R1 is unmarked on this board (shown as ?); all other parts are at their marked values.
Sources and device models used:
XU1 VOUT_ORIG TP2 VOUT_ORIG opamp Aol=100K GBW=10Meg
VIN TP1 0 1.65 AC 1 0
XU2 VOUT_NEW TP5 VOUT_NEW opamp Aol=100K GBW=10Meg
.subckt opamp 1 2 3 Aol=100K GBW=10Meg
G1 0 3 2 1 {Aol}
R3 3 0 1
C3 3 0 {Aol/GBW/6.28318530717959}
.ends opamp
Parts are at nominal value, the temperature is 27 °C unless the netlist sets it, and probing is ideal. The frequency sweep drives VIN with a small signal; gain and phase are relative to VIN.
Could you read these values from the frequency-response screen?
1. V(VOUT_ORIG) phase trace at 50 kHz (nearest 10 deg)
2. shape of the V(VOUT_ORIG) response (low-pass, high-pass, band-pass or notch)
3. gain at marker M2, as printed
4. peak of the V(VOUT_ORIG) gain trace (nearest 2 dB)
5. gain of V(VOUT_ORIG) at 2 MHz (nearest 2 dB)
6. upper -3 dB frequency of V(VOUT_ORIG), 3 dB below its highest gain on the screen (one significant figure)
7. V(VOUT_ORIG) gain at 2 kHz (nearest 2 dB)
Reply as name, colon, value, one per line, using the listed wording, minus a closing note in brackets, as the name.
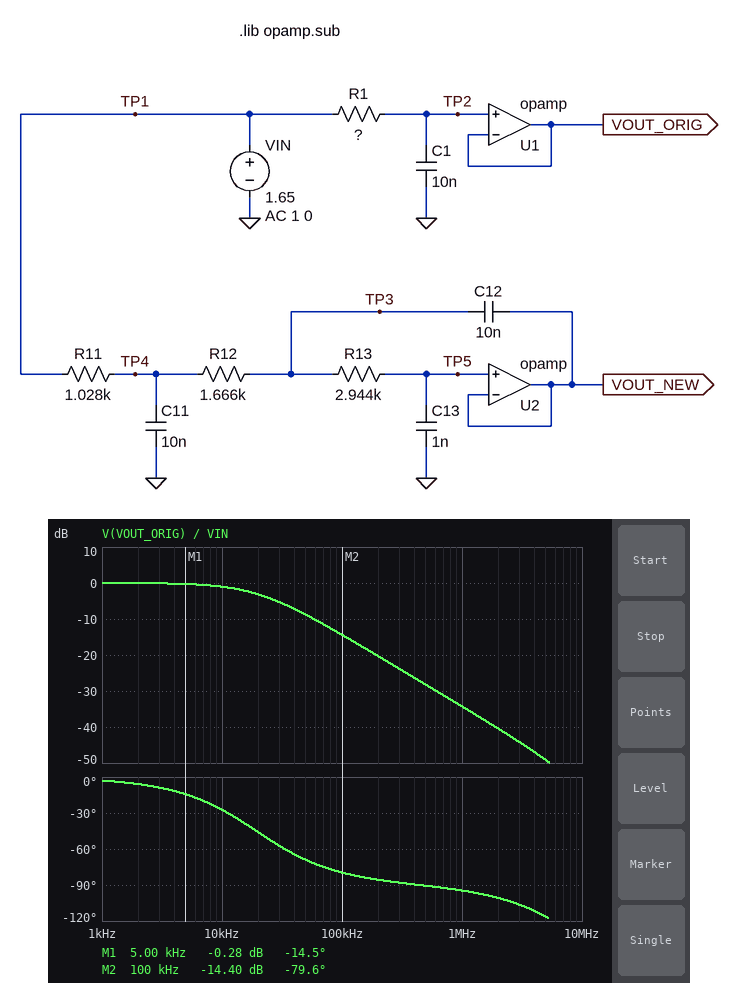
V(VOUT_ORIG) phase trace at 50 kHz: -70 deg
shape of the V(VOUT_ORIG) response: low-pass
gain at marker M2, as printed: -14.40 dB
peak of the V(VOUT_ORIG) gain trace: 0 dB
gain of V(VOUT_ORIG) at 2 MHz: -40 dB
upper -3 dB frequency of V(VOUT_ORIG), 3 dB below its highest gain on the screen: 20 kHz
V(VOUT_ORIG) gain at 2 kHz: 0 dB
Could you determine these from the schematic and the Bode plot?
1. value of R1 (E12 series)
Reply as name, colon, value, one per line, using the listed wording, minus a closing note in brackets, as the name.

value of R1: 820 Ω
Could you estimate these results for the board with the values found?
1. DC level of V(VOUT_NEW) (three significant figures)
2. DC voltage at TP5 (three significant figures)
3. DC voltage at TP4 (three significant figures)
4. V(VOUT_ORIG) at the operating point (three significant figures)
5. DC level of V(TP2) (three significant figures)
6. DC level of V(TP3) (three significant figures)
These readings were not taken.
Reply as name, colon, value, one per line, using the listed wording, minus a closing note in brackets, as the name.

DC level of V(VOUT_NEW): 1.65 V
DC voltage at TP5: 1.65 V
DC voltage at TP4: 1.65 V
V(VOUT_ORIG) at the operating point: 1.65 V
DC level of V(TP2): 1.65 V
DC level of V(TP3): 1.65 V
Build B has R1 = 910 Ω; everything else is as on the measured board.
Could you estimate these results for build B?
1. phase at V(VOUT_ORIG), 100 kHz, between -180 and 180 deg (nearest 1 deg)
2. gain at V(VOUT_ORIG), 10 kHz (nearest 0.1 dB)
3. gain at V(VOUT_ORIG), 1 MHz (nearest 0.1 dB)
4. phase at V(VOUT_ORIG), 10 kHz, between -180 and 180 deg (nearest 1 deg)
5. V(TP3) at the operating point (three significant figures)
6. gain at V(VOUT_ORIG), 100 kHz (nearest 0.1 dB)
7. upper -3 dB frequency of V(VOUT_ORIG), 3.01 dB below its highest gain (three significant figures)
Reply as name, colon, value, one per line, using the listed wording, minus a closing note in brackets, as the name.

phase at V(VOUT_ORIG), 100 kHz, between -180 and 180 deg: -81 deg
gain at V(VOUT_ORIG), 10 kHz: -1.2 dB
gain at V(VOUT_ORIG), 1 MHz: -35.2 dB
phase at V(VOUT_ORIG), 10 kHz, between -180 and 180 deg: -30 deg
V(TP3) at the operating point: 1.65 V
gain at V(VOUT_ORIG), 100 kHz: -15.3 dB
upper -3 dB frequency of V(VOUT_ORIG), 3.01 dB below its highest gain: 17.5 kHz
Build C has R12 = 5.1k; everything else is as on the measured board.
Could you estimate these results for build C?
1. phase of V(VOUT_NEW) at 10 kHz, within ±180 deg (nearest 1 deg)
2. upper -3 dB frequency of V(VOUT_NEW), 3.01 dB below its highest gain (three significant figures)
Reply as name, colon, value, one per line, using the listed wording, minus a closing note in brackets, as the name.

phase of V(VOUT_NEW) at 10 kHz, within ±180 deg: -93 deg
upper -3 dB frequency of V(VOUT_NEW), 3.01 dB below its highest gain: 13.7 kHz
